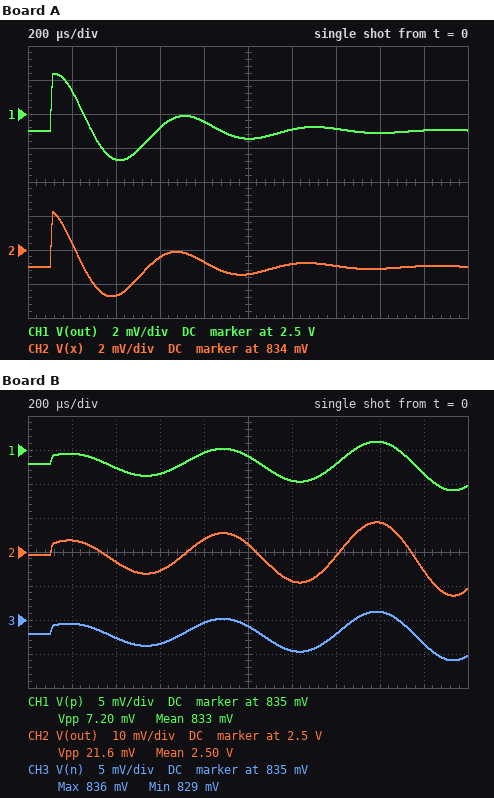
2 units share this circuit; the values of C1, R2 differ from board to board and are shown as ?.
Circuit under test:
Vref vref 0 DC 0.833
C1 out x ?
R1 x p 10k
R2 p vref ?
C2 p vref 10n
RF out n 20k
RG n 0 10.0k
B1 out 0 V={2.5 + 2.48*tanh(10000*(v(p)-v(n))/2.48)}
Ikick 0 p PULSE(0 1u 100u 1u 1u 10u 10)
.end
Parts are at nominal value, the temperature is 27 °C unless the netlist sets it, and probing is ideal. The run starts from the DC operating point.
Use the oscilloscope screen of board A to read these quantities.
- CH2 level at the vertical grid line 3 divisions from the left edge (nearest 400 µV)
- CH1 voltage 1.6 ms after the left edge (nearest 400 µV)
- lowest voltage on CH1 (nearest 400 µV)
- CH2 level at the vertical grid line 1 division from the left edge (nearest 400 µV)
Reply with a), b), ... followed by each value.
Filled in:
a) 833.6 mV
b) 2.4988 V
c) 2.4972 V
d) 834.4 mV
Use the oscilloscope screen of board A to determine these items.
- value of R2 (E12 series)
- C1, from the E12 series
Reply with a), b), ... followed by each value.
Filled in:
a) 5.6 kΩ
b) 15 nF
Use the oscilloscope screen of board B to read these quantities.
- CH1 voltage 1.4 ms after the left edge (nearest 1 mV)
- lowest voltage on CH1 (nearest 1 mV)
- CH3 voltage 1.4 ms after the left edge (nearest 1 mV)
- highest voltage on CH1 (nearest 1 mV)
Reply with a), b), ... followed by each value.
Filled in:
a) 833 mV
b) 829 mV
c) 833 mV
d) 836 mV
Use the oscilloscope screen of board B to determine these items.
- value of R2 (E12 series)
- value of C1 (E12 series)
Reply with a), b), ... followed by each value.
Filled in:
a) 8.2 kΩ
b) 15 nF
